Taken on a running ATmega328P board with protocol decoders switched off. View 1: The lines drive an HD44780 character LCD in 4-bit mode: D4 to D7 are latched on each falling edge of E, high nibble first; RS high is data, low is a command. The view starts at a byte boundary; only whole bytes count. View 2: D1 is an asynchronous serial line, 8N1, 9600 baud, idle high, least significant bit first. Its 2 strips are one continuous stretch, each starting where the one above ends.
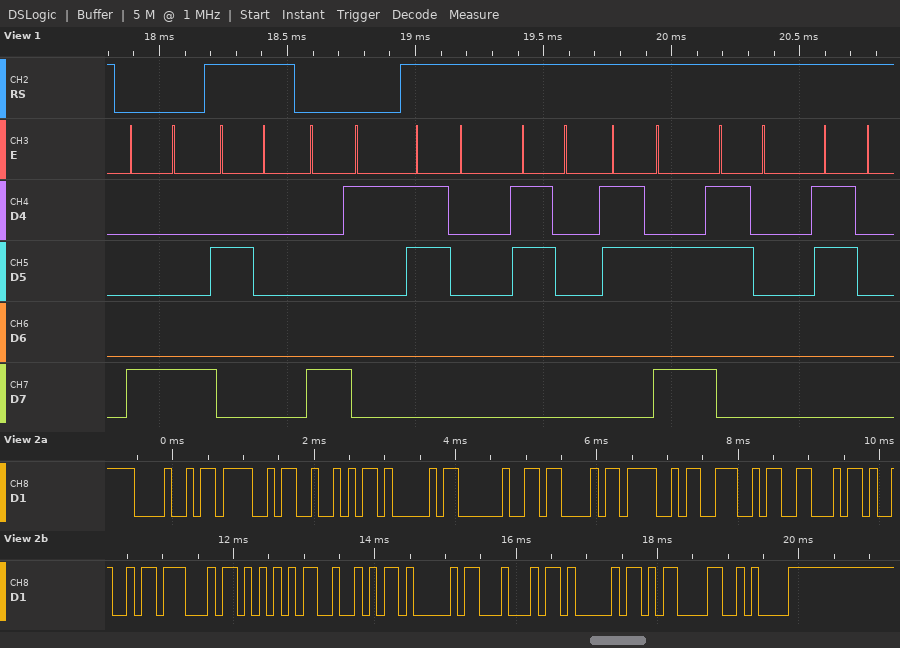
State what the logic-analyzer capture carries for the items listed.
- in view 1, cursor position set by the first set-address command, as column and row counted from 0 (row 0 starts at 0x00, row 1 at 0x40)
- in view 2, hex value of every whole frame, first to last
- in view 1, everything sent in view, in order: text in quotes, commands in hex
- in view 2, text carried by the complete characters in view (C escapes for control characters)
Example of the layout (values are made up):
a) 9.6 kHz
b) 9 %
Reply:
a) column 8, row 0
b) 48 4F 52 41 20 43 4F 4E 46 49 47 55 52 41 44 41 0D 0A
c) 0x88 " " 0x81 "00:00"
d) "HORA CONFIGURADA\r\n"
